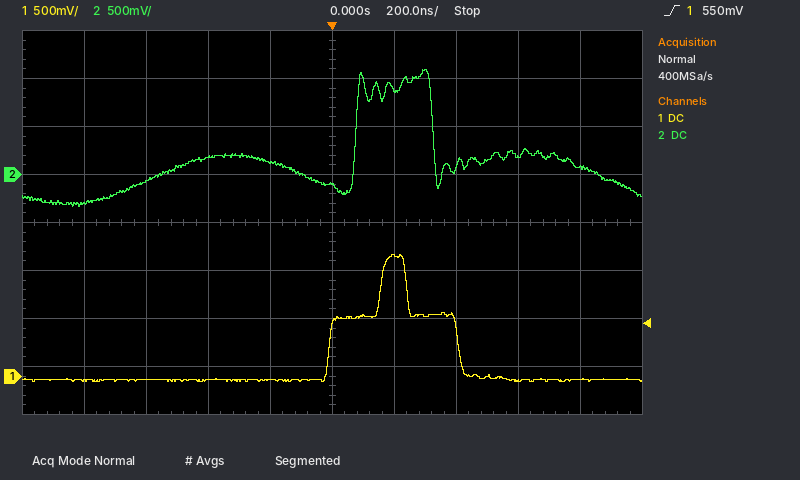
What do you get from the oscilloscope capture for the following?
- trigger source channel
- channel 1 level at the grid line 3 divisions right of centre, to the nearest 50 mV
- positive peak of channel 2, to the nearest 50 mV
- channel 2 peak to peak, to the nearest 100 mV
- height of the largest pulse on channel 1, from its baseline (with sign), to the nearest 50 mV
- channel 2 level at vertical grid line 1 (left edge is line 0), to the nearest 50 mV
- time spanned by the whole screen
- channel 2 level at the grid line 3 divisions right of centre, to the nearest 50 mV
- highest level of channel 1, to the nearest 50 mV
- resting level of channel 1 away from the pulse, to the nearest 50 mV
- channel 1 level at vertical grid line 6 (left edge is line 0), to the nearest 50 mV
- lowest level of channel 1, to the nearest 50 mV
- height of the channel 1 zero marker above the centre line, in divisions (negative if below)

channel 1
-50 mV
1.10 V
1.40 V
+1.30 V
-300 mV
2 µs
200 mV
1.25 V
-50 mV
1.25 V
-50 mV
-3.2 div
